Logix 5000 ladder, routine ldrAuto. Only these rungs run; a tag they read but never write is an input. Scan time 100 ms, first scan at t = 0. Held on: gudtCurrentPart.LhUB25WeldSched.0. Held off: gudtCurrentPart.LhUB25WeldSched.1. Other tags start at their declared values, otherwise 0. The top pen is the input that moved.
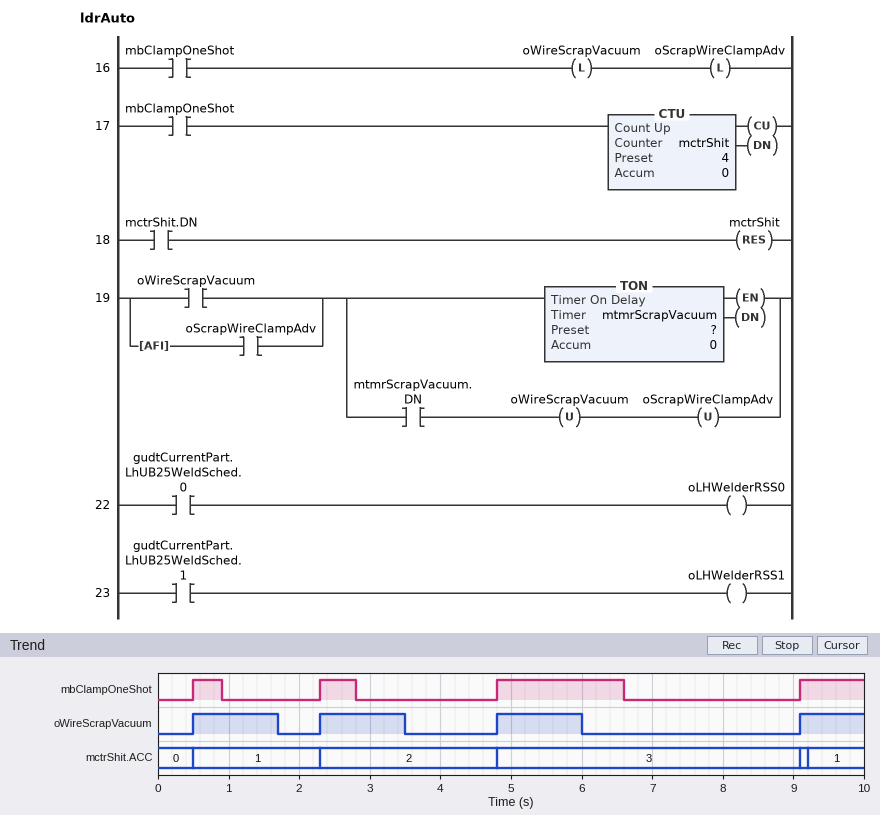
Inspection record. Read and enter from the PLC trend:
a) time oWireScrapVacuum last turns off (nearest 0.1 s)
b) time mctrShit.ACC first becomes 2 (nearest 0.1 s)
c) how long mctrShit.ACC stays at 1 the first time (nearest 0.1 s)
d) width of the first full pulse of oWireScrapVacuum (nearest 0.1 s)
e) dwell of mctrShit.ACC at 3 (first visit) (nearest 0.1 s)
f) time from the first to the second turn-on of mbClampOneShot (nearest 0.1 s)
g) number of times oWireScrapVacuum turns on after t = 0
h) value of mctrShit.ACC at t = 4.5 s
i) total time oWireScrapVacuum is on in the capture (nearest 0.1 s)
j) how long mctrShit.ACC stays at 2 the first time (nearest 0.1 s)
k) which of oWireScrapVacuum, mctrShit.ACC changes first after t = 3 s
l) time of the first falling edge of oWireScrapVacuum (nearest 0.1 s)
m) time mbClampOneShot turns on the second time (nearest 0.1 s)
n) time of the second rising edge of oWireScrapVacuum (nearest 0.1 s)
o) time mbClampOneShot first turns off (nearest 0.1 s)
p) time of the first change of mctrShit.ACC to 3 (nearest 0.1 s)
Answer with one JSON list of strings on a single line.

["6.0 s", "2.3 s", "1.8 s", "1.2 s", "4.3 s", "1.8 s", "4", "2", "4.5 s", "2.5 s", "oWireScrapVacuum", "1.7 s", "2.3 s", "2.3 s", "0.9 s", "4.8 s"]
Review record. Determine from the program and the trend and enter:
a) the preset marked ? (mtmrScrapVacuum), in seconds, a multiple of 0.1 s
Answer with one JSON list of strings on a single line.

["1.2 s"]
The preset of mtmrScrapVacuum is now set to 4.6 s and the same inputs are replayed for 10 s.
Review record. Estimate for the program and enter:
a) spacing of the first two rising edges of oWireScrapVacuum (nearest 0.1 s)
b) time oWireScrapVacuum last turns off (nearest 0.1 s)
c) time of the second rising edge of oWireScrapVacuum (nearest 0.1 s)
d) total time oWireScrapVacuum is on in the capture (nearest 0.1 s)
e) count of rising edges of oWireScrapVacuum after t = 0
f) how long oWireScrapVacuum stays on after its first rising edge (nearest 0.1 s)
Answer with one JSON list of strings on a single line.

["8.6 s", "5.1 s", "9.1 s", "5.5 s", "2", "4.6 s"]
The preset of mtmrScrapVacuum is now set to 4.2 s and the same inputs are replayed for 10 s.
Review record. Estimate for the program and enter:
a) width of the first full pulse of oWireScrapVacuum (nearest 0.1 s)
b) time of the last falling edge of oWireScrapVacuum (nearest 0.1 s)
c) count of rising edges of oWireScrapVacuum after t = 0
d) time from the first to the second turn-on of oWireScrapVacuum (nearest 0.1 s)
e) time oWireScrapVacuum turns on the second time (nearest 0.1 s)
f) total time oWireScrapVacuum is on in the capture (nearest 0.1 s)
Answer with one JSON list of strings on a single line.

["4.2 s", "4.7 s", "2", "8.6 s", "9.1 s", "5.1 s"]
